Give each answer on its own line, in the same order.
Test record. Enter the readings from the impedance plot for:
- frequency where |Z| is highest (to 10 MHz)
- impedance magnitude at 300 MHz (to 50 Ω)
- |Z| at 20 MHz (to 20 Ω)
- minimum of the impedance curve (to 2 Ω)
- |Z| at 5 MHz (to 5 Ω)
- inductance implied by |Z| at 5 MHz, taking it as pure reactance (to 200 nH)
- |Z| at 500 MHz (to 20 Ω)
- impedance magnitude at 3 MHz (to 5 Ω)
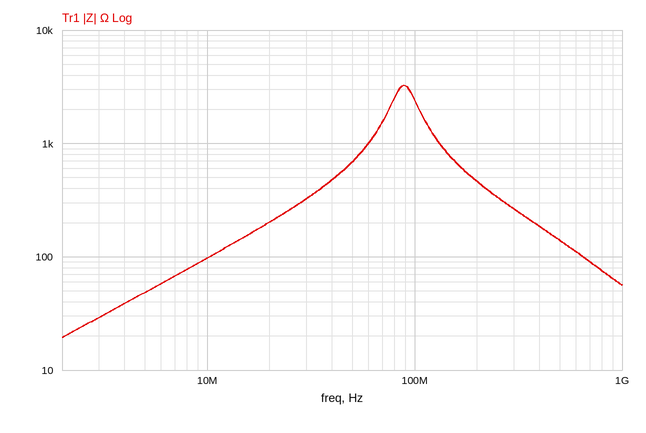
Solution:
90 MHz
250 Ω
200 Ω
20 Ω
50 Ω
1.6 µH
140 Ω
30 Ω
